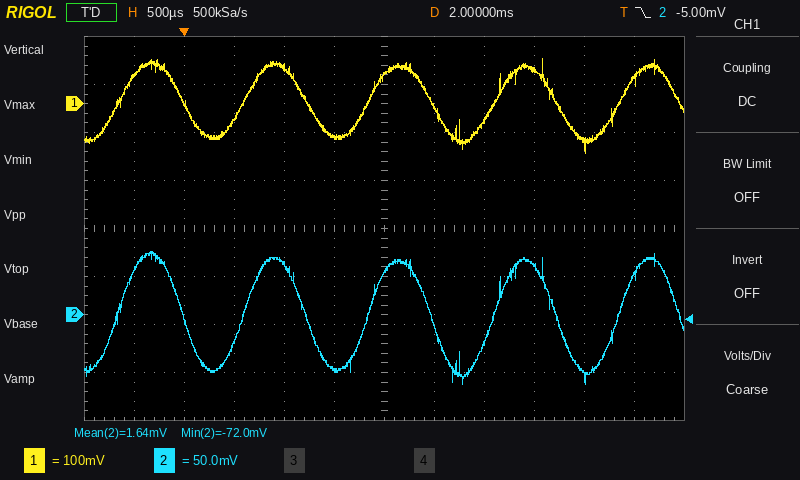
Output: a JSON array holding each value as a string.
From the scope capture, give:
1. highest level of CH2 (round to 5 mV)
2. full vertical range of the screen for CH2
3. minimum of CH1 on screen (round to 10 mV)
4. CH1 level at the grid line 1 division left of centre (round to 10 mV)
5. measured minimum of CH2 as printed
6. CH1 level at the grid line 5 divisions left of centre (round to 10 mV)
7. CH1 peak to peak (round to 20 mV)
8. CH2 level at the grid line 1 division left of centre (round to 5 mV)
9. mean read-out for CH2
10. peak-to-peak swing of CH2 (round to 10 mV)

["65 mV", "400 mV", "-100 mV", "-70 mV", "-72.0 mV", "60 mV", "200 mV", "-55 mV", "1.64 mV", "140 mV"]
